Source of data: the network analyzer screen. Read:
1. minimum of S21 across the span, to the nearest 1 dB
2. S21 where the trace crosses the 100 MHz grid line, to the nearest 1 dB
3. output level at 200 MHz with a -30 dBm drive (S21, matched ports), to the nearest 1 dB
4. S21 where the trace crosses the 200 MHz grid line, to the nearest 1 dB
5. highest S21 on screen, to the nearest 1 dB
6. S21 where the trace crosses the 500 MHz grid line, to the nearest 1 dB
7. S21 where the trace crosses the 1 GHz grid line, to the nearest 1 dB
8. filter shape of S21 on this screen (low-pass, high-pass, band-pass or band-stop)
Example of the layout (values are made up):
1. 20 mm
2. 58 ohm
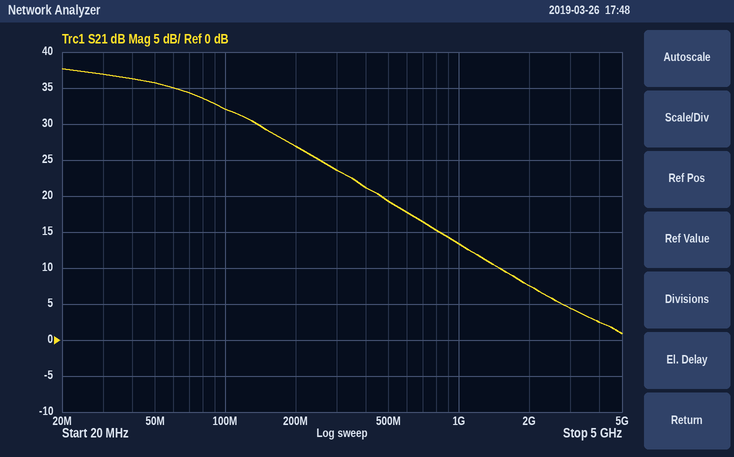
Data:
1. 1 dB
2. 32 dB
3. -3 dBm
4. 27 dB
5. 38 dB
6. 19 dB
7. 13 dB
8. low-pass
